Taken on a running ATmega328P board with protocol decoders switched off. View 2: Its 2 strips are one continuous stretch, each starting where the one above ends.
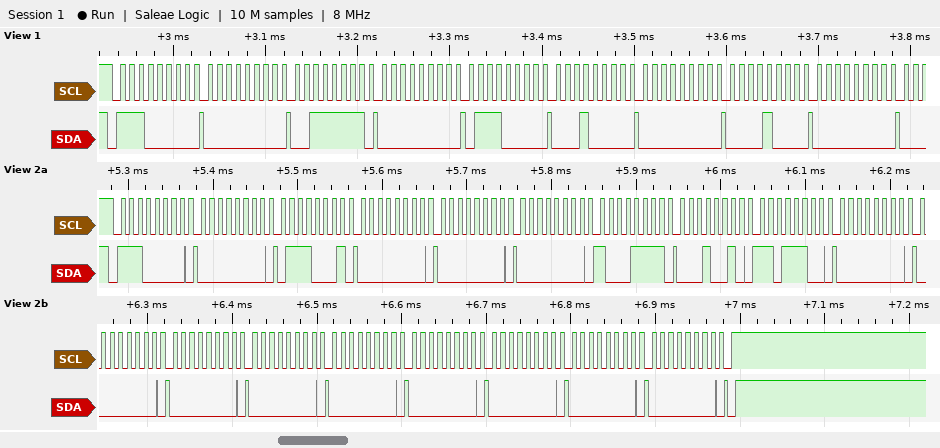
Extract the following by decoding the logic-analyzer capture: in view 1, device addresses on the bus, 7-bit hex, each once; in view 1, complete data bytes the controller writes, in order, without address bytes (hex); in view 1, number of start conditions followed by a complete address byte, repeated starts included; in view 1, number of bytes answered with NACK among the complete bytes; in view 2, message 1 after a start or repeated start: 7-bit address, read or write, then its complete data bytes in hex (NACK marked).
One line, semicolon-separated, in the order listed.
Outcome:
0x70; 00 3F 00 70 10 00 08 00; 1; 0; 0x70 write: 00 71 00 00 00 8F 12 DC 00 00 00 00 00 00 00 00 00
